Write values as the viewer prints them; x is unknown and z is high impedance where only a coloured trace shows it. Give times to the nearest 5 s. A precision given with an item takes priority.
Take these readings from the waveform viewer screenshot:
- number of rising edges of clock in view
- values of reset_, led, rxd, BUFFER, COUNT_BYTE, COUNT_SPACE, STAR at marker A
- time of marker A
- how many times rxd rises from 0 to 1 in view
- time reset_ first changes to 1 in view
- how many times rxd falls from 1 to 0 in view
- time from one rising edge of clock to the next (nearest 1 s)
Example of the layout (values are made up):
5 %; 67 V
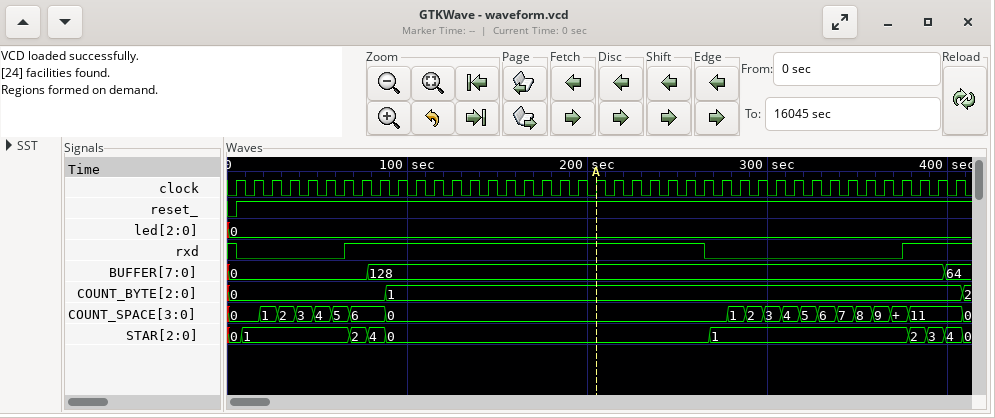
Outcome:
41; reset_=1, led=0, rxd=1, BUFFER=128, COUNT_BYTE=1, COUNT_SPACE=0, STAR=0; 205 s; 2; 5 s; 2; 10 s
